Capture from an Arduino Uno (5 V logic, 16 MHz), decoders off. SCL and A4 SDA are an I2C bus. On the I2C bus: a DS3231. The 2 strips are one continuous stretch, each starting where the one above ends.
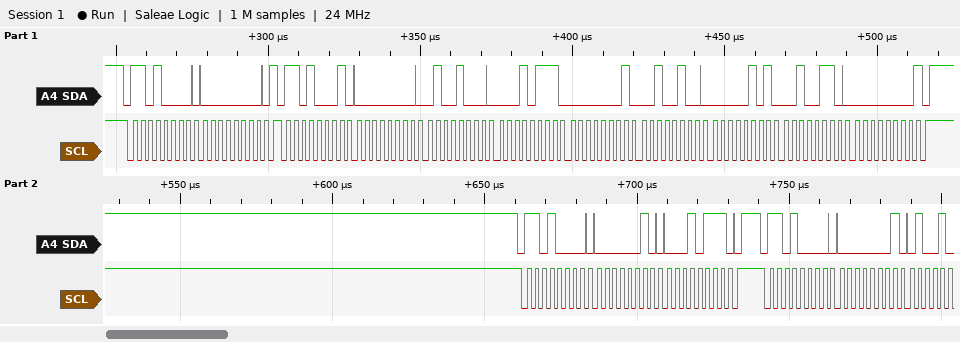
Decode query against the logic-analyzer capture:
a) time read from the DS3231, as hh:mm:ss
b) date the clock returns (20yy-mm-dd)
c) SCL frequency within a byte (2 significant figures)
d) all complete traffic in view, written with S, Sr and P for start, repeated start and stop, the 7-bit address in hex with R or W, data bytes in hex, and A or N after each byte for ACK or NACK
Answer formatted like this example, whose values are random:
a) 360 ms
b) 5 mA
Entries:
a) 17:48:00
b) 2026-05-24
c) 400 kHz
d) S 68W A 00 A Sr 68R A 00 A 48 A 17 A 01 A 24 A 05 A 26 A 00 N P S 68W A 02 A 17 A P S 68W A 01 A
